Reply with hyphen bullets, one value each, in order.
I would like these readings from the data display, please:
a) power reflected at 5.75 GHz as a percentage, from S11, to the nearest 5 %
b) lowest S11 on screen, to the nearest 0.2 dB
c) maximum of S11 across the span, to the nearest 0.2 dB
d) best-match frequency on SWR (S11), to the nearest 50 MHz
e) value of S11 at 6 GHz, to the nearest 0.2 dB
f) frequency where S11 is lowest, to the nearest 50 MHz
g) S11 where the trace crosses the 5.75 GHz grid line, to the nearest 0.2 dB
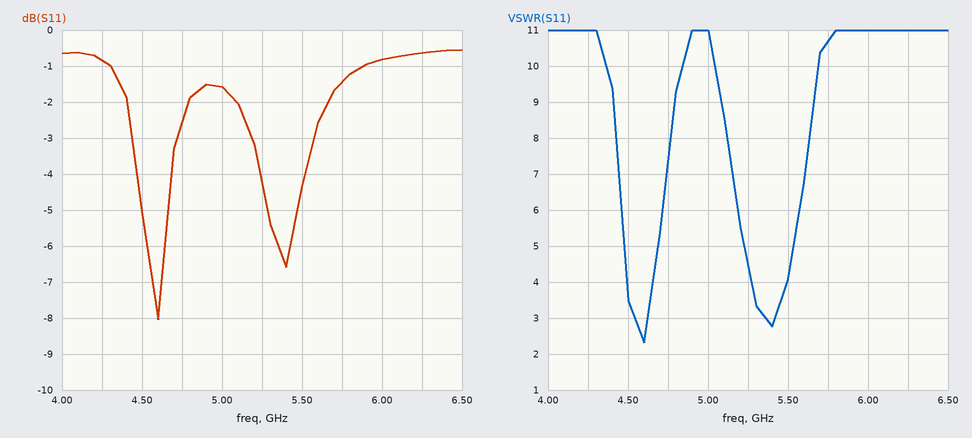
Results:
- 70 %
- -8.0 dB
- -0.6 dB
- 4.60 GHz
- -0.8 dB
- 4.60 GHz
- -1.4 dB
